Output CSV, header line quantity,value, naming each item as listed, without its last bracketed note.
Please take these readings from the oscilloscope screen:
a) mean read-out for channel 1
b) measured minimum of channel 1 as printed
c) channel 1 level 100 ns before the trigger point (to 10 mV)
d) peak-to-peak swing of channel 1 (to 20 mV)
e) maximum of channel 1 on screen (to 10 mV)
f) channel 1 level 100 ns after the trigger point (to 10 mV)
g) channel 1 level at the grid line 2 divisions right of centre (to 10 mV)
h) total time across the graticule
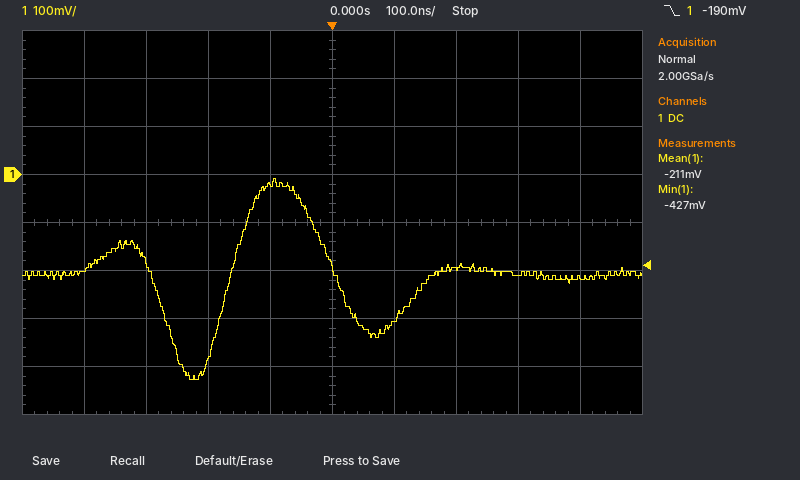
quantity,value
mean read-out for channel 1,-211 mV
measured minimum of channel 1 as printed,-427 mV
channel 1 level 100 ns before the trigger point,-20 mV
peak-to-peak swing of channel 1,420 mV
maximum of channel 1 on screen,-10 mV
channel 1 level 100 ns after the trigger point,-310 mV
channel 1 level at the grid line 2 divisions right of centre,-200 mV
total time across the graticule,1 µs
